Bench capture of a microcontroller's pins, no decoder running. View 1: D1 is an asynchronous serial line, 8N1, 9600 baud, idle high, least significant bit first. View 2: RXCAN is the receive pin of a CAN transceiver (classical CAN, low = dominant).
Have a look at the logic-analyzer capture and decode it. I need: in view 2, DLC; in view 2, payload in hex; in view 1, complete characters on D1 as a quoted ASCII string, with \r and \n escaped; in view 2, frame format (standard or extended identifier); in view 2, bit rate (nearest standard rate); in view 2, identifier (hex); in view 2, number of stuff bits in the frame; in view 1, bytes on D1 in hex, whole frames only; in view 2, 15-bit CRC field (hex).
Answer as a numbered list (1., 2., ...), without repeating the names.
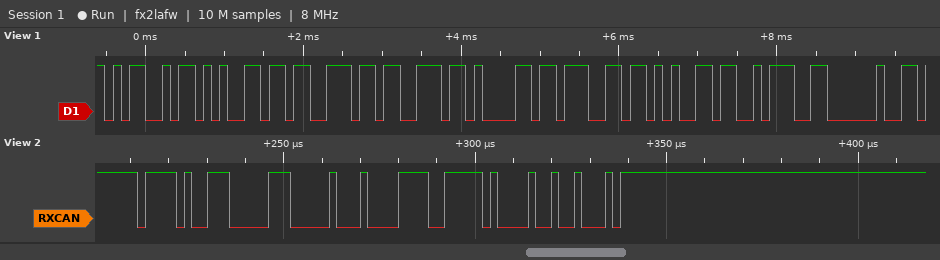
1. 3
2. 00 87 9F
3. "Message: "
4. standard
5. 500 kbit/s
6. 0x7A7
7. 3
8. 0x4D 0x65 0x73 0x73 0x61 0x67 0x65 0x3A 0x20
9. 0x4248
